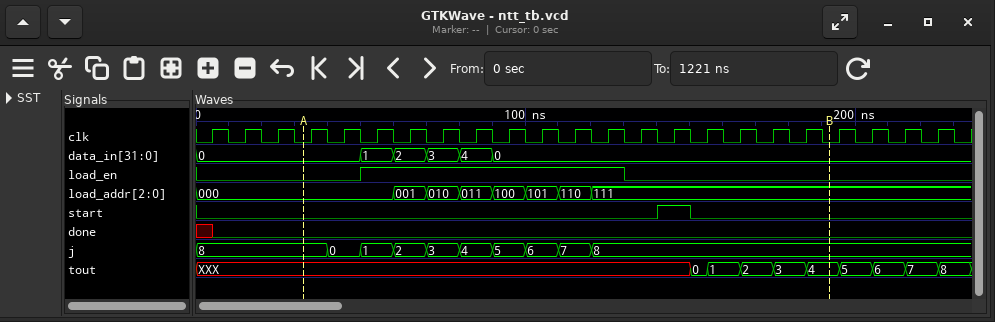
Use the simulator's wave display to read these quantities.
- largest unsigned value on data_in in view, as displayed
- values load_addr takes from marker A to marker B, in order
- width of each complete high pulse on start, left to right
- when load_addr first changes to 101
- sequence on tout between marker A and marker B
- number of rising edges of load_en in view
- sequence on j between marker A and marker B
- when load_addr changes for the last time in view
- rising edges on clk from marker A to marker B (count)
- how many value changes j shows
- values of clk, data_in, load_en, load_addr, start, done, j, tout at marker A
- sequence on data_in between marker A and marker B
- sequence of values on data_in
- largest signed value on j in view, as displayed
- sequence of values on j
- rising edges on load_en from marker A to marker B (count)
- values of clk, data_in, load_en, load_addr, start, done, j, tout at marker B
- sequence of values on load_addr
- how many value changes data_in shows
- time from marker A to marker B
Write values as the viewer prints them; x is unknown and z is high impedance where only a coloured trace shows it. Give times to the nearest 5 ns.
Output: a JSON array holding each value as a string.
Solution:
["4", "000, 001, 010, 011, 100, 101, 110, 111", "10 ns", "100 ns", "XXX, 0, 1, 2, 3, 4", "1", "8, 0, 1, 2, 3, 4, 5, 6, 7, 8", "120 ns", "16", "9", "clk=0, data_in=0, load_en=0, load_addr=000, start=0, done=0, j=8, tout=XXX", "0, 1, 2, 3, 4, 0", "0, 1, 2, 3, 4, 0", "8", "8, 0, 1, 2, 3, 4, 5, 6, 7, 8", "1", "clk=0, data_in=0, load_en=0, load_addr=111, start=0, done=0, j=8, tout=4", "000, 001, 010, 011, 100, 101, 110, 111", "5", "160 ns"]
